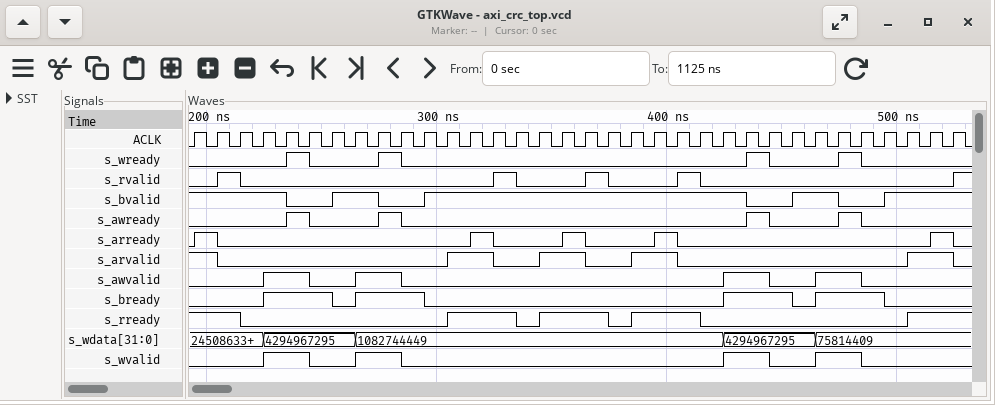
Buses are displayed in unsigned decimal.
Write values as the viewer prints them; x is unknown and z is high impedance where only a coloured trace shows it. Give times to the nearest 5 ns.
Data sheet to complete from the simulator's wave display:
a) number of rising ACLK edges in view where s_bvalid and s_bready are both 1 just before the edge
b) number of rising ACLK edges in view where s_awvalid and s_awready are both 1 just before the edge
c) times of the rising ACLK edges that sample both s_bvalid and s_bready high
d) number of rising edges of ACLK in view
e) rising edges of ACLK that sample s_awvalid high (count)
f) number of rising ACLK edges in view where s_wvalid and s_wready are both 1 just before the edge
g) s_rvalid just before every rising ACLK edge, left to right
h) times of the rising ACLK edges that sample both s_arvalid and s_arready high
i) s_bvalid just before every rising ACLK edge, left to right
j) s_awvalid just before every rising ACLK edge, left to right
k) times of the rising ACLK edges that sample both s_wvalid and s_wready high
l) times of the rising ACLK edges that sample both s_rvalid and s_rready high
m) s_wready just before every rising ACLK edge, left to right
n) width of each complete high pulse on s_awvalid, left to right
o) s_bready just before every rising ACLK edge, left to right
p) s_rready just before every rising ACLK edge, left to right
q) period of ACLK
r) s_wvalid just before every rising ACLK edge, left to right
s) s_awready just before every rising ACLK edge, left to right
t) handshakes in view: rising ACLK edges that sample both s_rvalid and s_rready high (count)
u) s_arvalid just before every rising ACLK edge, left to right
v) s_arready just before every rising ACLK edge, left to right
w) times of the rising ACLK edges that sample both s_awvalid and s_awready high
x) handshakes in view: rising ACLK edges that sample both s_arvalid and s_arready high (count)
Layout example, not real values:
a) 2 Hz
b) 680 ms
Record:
a) 4
b) 4
c) 235 ns, 275 ns, 435 ns, 475 ns
d) 34
e) 8
f) 4
g) 0 0 1 0 0 0 0 0 0 0 0 0 0 0 1 0 0 0 1 0 0 0 1 0 0 0 0 0 0 0 0 0 0 0
h) 205 ns, 325 ns, 365 ns, 405 ns, 525 ns
i) 1 1 1 1 1 0 0 1 1 0 0 1 1 1 1 1 1 1 1 1 1 1 1 1 1 0 0 1 1 0 0 1 1 1
j) 0 0 0 0 1 1 0 0 1 1 0 0 0 0 0 0 0 0 0 0 0 0 0 0 1 1 0 0 1 1 0 0 0 0
k) 245 ns, 285 ns, 445 ns, 485 ns
l) 215 ns, 335 ns, 375 ns, 415 ns
m) 0 0 0 0 0 1 0 0 0 1 0 0 0 0 0 0 0 0 0 0 0 0 0 0 0 1 0 0 0 1 0 0 0 0
n) 20 ns, 20 ns, 20 ns, 20 ns
o) 0 0 0 0 1 1 1 0 1 1 1 0 0 0 0 0 0 0 0 0 0 0 0 0 1 1 1 0 1 1 1 0 0 0
p) 1 1 1 0 0 0 0 0 0 0 0 0 1 1 1 0 1 1 1 0 1 1 1 0 0 0 0 0 0 0 0 0 1 1
q) 10 ns
r) 0 0 0 0 1 1 0 0 1 1 0 0 0 0 0 0 0 0 0 0 0 0 0 0 1 1 0 0 1 1 0 0 0 0
s) 0 0 0 0 0 1 0 0 0 1 0 0 0 0 0 0 0 0 0 0 0 0 0 0 0 1 0 0 0 1 0 0 0 0
t) 4
u) 1 1 0 0 0 0 0 0 0 0 0 0 1 1 0 0 1 1 0 0 1 1 0 0 0 0 0 0 0 0 0 0 1 1
v) 0 1 0 0 0 0 0 0 0 0 0 0 0 1 0 0 0 1 0 0 0 1 0 0 0 0 0 0 0 0 0 0 0 1
w) 245 ns, 285 ns, 445 ns, 485 ns
x) 5
